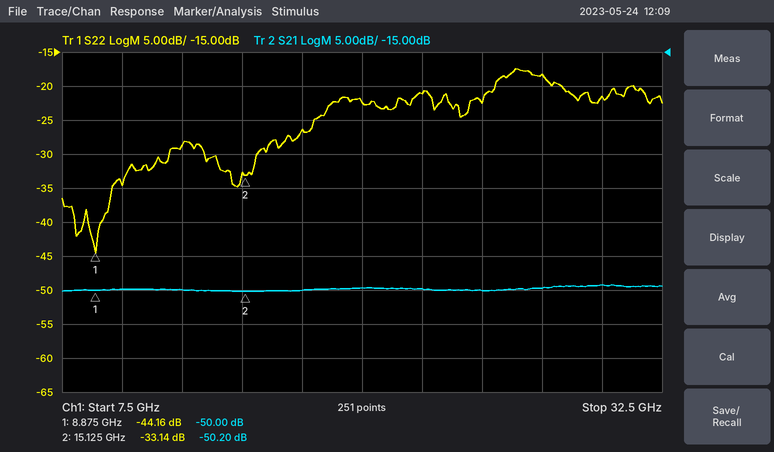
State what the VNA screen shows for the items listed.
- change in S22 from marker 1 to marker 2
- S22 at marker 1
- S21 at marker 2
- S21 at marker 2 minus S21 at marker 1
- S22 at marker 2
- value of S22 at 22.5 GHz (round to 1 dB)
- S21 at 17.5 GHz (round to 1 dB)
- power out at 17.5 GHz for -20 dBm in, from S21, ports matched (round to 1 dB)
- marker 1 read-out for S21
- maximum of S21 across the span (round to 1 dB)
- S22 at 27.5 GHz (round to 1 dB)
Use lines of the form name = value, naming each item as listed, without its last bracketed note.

change in S22 from marker 1 to marker 2 = 11.02 dB
S22 at marker 1 = -44.16 dB
S21 at marker 2 = -50.20 dB
S21 at marker 2 minus S21 at marker 1 = -0.20 dB
S22 at marker 2 = -33.14 dB
value of S22 at 22.5 GHz = -21 dB
S21 at 17.5 GHz = -50 dB
power out at 17.5 GHz for -20 dBm in, from S21, ports matched = -70 dBm
marker 1 read-out for S21 = -50.00 dB
maximum of S21 across the span = -49 dB
S22 at 27.5 GHz = -18 dB
